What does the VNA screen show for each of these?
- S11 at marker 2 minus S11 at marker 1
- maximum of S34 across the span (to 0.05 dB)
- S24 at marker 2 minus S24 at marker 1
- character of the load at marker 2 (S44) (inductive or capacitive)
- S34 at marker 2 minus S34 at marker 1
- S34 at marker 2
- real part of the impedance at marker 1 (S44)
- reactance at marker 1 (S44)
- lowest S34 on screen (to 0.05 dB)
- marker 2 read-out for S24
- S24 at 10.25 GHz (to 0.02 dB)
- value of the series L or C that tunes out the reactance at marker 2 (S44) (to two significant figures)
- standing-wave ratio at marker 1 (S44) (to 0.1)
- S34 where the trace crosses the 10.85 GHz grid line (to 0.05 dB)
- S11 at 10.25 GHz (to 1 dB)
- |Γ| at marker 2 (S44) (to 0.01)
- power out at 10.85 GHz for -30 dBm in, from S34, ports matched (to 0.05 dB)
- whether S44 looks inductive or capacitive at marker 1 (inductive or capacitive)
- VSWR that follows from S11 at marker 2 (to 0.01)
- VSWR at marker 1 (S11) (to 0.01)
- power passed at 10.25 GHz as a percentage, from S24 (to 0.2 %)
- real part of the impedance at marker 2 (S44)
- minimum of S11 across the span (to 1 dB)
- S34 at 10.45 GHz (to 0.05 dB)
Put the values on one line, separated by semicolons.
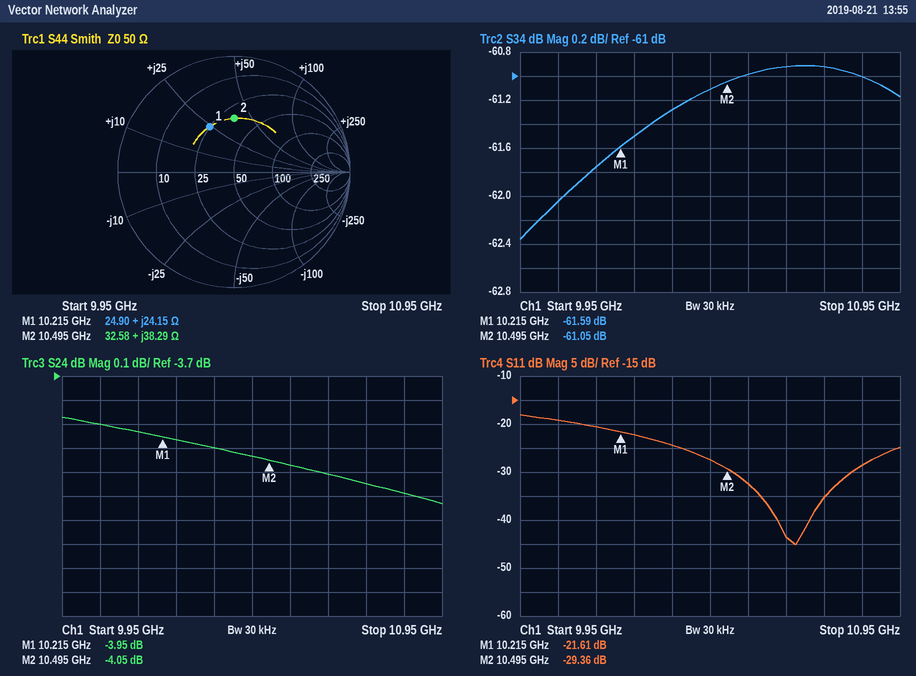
-7.75 dB; -60.90 dB; -0.10 dB; inductive; 0.54 dB; -61.05 dB; 24.90 Ω; +24.15 Ω; -62.35 dB; -4.05 dB; -3.96 dB; 400 fF; 2.6; -61.00 dB; -22 dB; 0.46; -91.00 dBm; inductive; 1.07; 1.18; 40.2 %; 32.58 Ω; -45 dB; -61.10 dB
